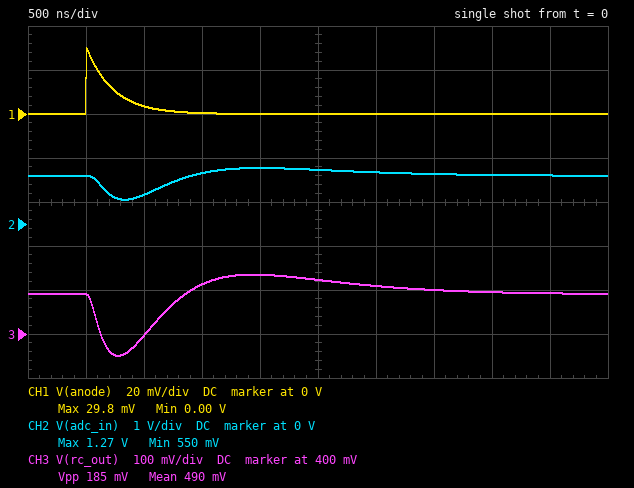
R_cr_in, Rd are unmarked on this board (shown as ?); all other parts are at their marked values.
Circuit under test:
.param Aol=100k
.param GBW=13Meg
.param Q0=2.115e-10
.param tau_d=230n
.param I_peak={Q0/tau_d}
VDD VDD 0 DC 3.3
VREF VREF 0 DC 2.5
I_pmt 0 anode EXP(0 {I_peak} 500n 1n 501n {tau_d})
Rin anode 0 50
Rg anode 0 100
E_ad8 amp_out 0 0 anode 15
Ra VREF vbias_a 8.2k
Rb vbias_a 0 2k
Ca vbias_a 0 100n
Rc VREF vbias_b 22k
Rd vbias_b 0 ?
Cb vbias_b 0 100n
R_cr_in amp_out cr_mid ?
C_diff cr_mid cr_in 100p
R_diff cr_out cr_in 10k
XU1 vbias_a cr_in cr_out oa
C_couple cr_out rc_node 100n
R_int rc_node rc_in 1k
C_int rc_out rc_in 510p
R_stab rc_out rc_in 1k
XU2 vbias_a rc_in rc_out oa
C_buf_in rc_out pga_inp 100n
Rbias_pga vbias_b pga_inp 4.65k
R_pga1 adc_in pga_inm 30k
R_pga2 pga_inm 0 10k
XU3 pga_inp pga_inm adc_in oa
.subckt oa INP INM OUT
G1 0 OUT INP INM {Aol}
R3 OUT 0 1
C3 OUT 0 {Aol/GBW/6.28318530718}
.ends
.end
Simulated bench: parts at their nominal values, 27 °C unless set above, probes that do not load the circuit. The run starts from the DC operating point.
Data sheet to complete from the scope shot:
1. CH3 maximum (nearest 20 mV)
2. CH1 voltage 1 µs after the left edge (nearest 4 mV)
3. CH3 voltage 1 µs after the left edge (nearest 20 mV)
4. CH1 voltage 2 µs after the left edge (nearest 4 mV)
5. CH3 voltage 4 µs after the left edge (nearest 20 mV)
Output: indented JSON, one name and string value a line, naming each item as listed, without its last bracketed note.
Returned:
{
  "CH3 maximum": "540 mV",
  "CH1 voltage 1 µs after the left edge": "4 mV",
  "CH3 voltage 1 µs after the left edge": "400 mV",
  "CH1 voltage 2 µs after the left edge": "0 V",
  "CH3 voltage 4 µs after the left edge": "500 mV"
}
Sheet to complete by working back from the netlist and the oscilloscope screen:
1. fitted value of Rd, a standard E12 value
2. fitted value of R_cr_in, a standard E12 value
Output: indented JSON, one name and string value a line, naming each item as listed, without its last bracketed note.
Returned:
{
  "fitted value of Rd, a standard E12 value": "2.7 kΩ",
  "fitted value of R_cr_in, a standard E12 value": "5.6 kΩ"
}
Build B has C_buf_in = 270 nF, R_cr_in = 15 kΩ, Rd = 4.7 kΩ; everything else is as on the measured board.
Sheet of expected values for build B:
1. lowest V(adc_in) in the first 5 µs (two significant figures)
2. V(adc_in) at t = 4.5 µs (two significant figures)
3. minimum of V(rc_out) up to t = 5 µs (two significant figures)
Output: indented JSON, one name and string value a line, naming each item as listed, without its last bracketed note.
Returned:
{
  "lowest V(adc_in) in the first 5 µs": "1.5 V",
  "V(adc_in) at t = 4.5 µs": "1.8 V",
  "minimum of V(rc_out) up to t = 5 µs": "430 mV"
}
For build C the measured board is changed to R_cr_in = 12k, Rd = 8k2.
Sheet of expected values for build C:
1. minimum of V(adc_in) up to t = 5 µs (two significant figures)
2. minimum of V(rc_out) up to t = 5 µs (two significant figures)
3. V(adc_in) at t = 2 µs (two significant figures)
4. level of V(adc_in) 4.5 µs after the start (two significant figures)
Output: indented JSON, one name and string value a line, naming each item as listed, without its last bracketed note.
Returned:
{
  "minimum of V(adc_in) up to t = 5 µs": "2.4 V",
  "minimum of V(rc_out) up to t = 5 µs": "420 mV",
  "V(adc_in) at t = 2 µs": "2.8 V",
  "level of V(adc_in) 4.5 µs after the start": "2.7 V"
}
